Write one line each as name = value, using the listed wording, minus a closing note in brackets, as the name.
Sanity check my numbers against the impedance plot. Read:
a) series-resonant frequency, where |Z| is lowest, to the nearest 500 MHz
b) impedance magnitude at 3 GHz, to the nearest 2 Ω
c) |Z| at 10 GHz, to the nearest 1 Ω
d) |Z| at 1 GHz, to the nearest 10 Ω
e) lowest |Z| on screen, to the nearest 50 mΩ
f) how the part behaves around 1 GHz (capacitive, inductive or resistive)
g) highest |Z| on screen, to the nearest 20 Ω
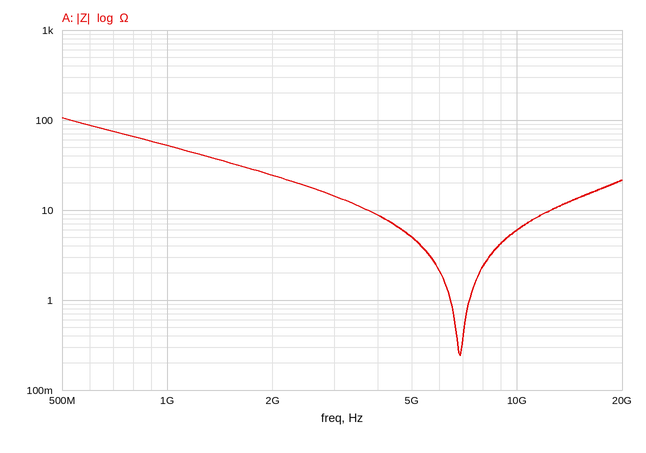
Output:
series-resonant frequency, where |Z| is lowest, to the nearest 500 MHz = 7.0 GHz
impedance magnitude at 3 GHz, to the nearest 2 Ω = 14 Ω
|Z| at 10 GHz, to the nearest 1 Ω = 6 Ω
|Z| at 1 GHz, to the nearest 10 Ω = 50 Ω
lowest |Z| on screen, to the nearest 50 mΩ = 250 mΩ
how the part behaves around 1 GHz = capacitive
highest |Z| on screen, to the nearest 20 Ω = 100 Ω
